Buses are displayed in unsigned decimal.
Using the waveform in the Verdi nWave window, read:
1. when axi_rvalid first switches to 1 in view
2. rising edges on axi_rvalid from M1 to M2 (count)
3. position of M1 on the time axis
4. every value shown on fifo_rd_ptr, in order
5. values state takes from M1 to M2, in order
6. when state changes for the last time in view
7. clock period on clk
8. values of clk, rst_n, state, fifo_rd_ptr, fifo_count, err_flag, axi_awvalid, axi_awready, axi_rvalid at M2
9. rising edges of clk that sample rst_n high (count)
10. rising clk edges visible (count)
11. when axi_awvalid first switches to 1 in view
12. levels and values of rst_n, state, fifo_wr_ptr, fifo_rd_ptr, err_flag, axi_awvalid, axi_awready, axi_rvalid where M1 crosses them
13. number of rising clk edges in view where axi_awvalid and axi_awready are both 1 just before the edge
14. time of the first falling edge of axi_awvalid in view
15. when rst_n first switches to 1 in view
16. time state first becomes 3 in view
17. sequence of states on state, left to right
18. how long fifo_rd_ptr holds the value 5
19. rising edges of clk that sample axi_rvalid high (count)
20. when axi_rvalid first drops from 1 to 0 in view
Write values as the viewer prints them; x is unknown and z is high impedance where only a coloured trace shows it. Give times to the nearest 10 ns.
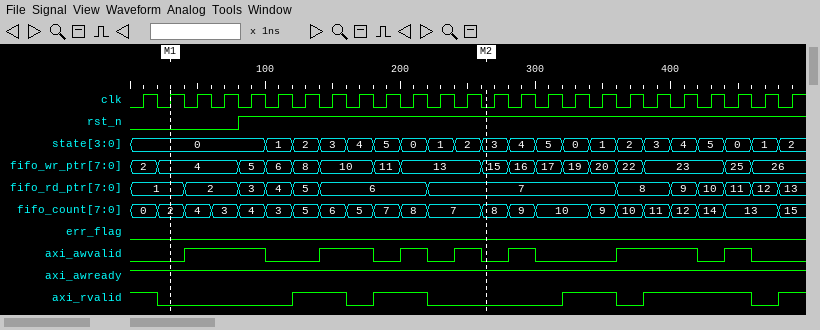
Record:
120 ns
2
30 ns
1, 2, 3, 4, 5, 6, 7, 8, 9, 10, 11, 12, 13
0, 1, 2, 3, 4, 5, 0, 1, 2, 3
480 ns
20 ns
clk=0, rst_n=1, state=3, fifo_rd_ptr=7, fifo_count=8, err_flag=0, axi_awvalid=0, axi_awready=1, axi_rvalid=0
21
25
40 ns
rst_n=0, state=0, fifo_wr_ptr=4, fifo_rd_ptr=1, err_flag=0, axi_awvalid=0, axi_awready=1, axi_rvalid=0
12
100 ns
80 ns
140 ns
0, 1, 2, 3, 4, 5, 0, 1, 2, 3, 4, 5, 0, 1, 2, 3, 4, 5, 0, 1, 2
20 ns
12
20 ns
